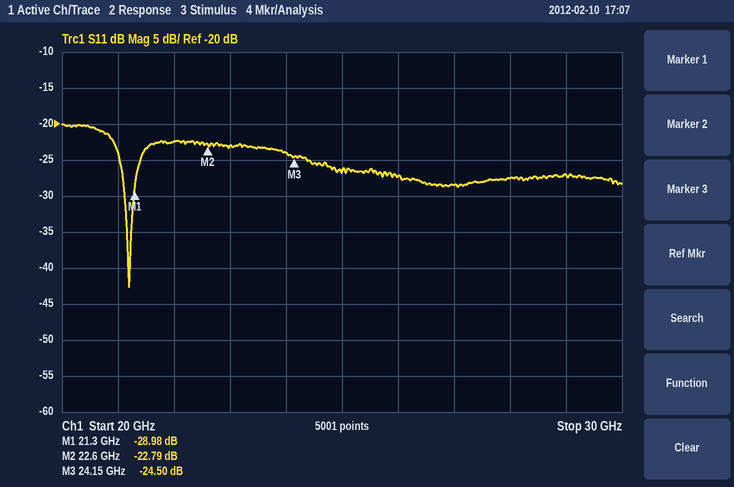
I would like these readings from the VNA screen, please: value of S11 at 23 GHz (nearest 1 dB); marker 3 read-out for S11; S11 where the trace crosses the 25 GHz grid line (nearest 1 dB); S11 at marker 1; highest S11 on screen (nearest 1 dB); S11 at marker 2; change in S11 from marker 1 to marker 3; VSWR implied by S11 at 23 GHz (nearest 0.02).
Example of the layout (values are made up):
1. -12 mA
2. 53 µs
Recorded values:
1. -23 dB
2. -24.50 dB
3. -27 dB
4. -28.98 dB
5. -20 dB
6. -22.79 dB
7. 4.48 dB
8. 1.16
